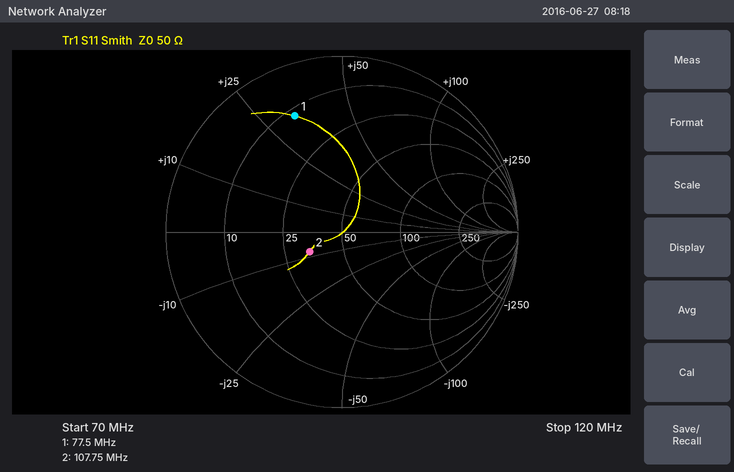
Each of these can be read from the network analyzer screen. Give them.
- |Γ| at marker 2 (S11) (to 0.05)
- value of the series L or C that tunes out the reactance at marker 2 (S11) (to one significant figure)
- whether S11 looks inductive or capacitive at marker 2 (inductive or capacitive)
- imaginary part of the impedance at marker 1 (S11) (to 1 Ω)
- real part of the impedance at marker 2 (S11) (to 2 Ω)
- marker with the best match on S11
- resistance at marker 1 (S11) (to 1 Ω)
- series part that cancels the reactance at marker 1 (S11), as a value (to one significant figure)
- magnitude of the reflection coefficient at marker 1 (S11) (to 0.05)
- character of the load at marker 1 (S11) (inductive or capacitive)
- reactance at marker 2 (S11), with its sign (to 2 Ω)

0.20
10 nH
capacitive
+32 Ω
34 Ω
marker 2
12 Ω
60 pF
0.70
inductive
-8 Ω
